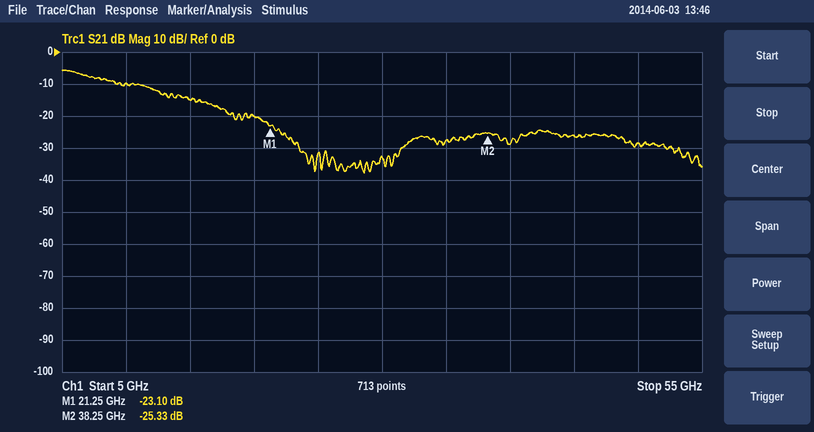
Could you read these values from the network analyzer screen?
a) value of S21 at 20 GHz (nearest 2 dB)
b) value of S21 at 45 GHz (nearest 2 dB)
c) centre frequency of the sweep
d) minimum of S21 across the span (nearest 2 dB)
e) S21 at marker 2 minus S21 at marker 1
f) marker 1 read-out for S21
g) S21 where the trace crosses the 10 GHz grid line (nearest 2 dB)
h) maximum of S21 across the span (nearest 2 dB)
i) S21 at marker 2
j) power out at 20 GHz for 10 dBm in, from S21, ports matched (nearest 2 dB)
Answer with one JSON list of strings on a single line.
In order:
["-20 dB", "-26 dB", "30 GHz", "-38 dB", "-2.23 dB", "-23.10 dB", "-10 dB", "-6 dB", "-25.33 dB", "-10 dBm"]
